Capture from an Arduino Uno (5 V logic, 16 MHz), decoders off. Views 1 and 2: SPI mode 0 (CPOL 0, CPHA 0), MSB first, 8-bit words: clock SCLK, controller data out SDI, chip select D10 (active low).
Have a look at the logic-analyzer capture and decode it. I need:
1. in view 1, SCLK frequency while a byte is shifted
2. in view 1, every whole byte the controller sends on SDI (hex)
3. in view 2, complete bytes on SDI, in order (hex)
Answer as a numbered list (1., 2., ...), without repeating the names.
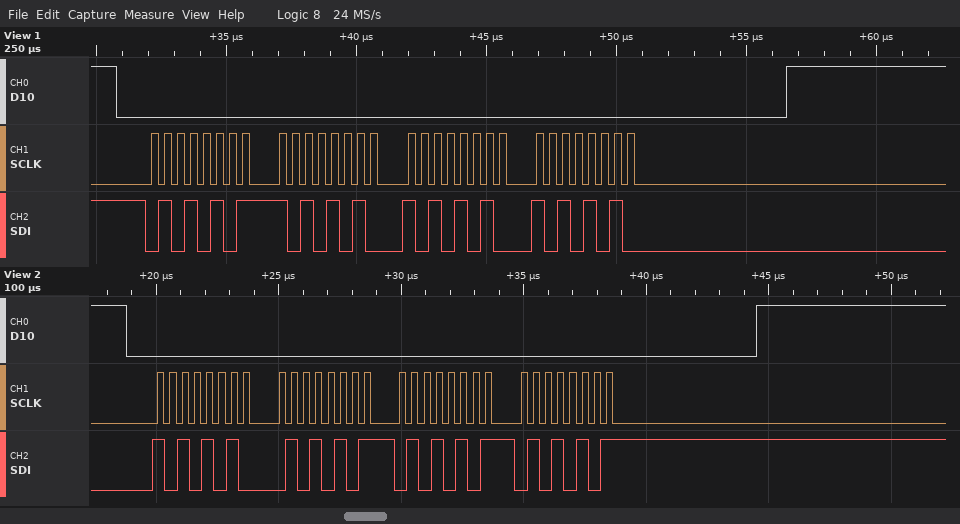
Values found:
1. 2 MHz
2. 55 AA AA AA
3. AA 55 55 55
